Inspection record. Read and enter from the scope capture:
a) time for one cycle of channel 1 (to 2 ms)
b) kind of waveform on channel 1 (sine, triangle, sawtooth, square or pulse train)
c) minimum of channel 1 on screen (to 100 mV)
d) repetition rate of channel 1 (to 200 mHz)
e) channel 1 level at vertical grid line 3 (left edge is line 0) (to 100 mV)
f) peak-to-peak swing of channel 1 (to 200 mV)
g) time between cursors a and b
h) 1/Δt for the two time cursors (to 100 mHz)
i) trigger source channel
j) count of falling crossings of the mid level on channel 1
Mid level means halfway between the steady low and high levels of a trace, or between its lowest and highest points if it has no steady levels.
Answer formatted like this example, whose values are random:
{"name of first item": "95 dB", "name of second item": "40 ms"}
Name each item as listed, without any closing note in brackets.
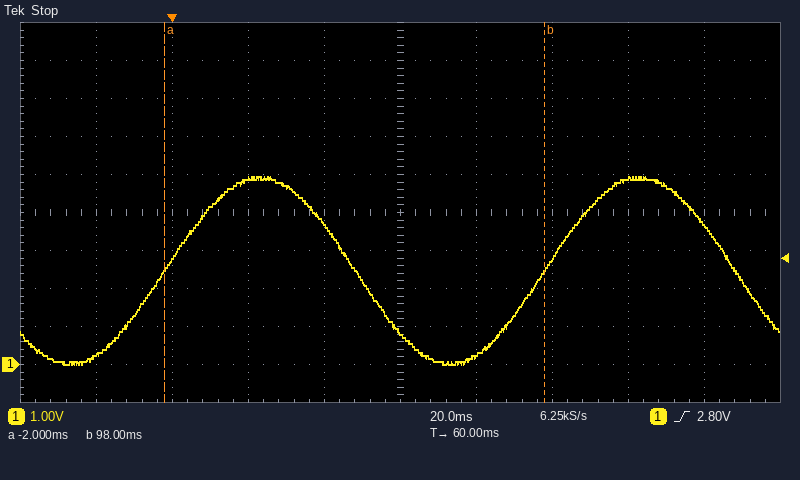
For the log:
{"time for one cycle of channel 1": "100 ms", "kind of waveform on channel 1": "sine", "minimum of channel 1 on screen": "0.0 V", "repetition rate of channel 1": "10.0 Hz", "channel 1 level at vertical grid line 3 (left edge is line 0)": "4.9 V", "peak-to-peak swing of channel 1": "5.0 V", "time between cursors a and b": "100 ms", "1/Δt for the two time cursors": "10.0 Hz", "trigger source channel": "channel 1", "count of falling crossings of the mid level on channel 1": "2"}
